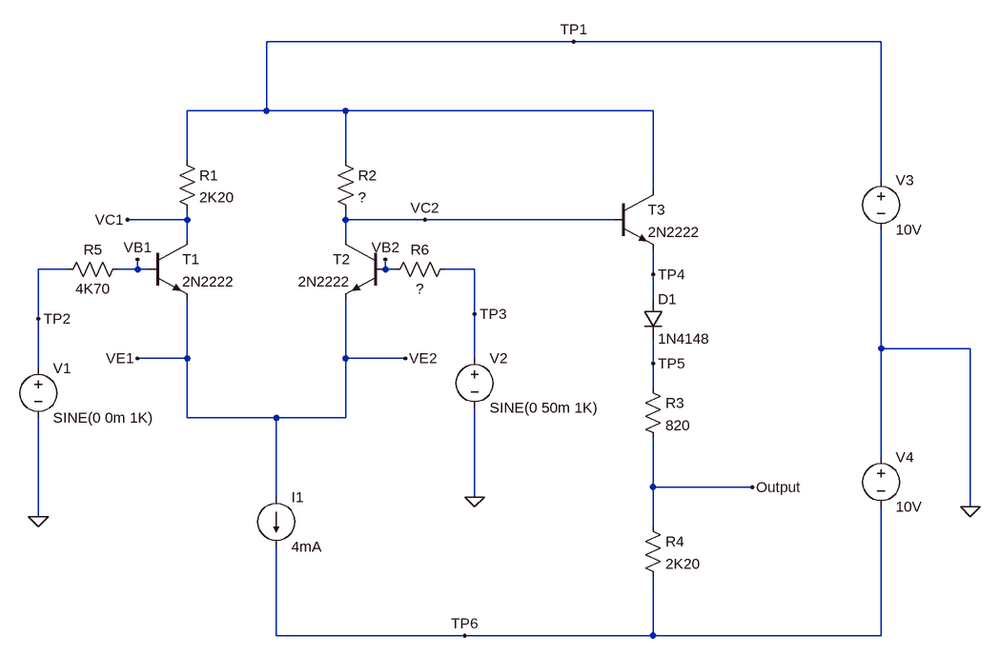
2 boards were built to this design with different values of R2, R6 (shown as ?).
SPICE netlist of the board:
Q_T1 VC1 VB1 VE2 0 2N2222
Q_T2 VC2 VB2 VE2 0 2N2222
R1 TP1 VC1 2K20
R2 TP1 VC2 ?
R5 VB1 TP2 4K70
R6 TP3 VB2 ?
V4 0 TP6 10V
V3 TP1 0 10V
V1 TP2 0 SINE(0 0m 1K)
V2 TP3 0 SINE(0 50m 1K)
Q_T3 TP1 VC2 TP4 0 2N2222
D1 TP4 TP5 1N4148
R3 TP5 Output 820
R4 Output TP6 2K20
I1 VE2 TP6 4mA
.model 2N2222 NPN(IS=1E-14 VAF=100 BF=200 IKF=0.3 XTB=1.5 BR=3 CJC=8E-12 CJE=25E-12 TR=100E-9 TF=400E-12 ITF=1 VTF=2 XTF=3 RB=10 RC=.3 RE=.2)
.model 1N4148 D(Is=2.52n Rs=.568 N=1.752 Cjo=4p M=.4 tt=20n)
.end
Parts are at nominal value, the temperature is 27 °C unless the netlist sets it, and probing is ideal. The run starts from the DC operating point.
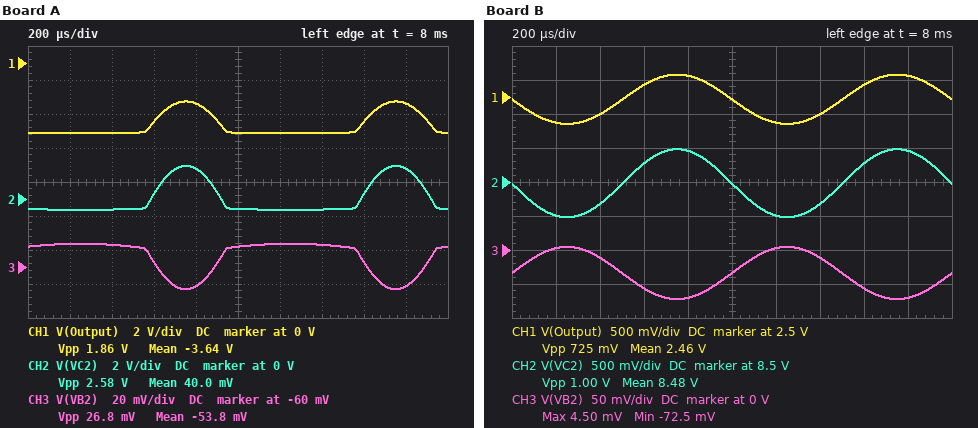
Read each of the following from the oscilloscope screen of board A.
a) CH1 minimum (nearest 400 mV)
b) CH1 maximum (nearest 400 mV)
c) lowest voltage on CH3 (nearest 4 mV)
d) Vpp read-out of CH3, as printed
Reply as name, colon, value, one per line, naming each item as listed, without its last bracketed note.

CH1 minimum: -4.0 V
CH1 maximum: -2.4 V
lowest voltage on CH3: -72 mV
Vpp read-out of CH3, as printed: 26.8 mV
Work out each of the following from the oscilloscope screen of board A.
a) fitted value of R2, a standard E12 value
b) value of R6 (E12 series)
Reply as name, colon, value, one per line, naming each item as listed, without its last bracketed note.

fitted value of R2, a standard E12 value: 5.6 kΩ
value of R6: 3.3 kΩ
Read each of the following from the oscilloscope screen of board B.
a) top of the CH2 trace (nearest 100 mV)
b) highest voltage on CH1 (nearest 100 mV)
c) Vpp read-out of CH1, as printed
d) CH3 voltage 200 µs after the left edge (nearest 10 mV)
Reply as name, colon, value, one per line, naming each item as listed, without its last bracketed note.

top of the CH2 trace: 9.0 V
highest voltage on CH1: 2.8 V
Vpp read-out of CH1, as printed: 725 mV
CH3 voltage 200 µs after the left edge: 0 V
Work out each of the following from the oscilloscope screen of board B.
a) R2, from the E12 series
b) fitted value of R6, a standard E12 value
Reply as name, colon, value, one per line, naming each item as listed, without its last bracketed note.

R2, from the E12 series: 680 Ω
fitted value of R6, a standard E12 value: 3.3 kΩ
